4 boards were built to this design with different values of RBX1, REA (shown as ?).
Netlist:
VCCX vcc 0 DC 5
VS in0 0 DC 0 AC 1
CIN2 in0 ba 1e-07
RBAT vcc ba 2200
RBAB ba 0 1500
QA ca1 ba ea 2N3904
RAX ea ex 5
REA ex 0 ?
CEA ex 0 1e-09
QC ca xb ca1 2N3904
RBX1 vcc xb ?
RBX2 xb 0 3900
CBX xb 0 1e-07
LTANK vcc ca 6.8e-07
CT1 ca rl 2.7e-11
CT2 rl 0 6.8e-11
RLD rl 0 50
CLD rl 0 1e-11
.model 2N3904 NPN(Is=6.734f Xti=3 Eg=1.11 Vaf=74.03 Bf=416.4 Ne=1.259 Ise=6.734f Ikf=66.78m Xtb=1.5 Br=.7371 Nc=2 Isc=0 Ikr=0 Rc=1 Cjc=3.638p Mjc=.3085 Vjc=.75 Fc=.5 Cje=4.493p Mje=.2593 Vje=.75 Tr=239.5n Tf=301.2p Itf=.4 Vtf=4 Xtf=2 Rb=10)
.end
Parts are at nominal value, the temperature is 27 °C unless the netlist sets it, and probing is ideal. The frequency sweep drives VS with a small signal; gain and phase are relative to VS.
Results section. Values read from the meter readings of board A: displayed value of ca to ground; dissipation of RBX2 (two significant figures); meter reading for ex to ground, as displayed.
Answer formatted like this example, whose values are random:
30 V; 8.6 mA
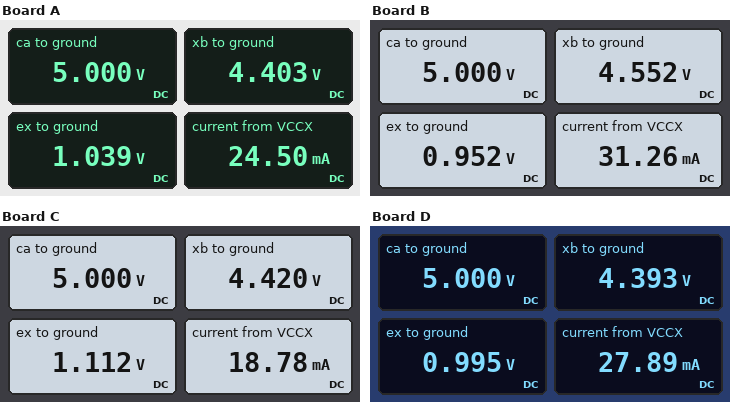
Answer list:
5.000 V; 5.0 mW; 1.039 V
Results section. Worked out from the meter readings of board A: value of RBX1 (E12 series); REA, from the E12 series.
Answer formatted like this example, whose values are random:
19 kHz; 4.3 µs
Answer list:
470 Ω; 47 Ω
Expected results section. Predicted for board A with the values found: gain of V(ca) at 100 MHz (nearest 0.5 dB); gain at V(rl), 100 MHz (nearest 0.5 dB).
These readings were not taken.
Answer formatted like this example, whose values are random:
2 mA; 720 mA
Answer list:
20.5 dB; 8.5 dB
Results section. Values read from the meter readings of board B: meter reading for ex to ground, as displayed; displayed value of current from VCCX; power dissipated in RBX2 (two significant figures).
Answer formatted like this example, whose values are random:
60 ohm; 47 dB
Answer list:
0.952 V; 31.26 mA; 5.3 mW
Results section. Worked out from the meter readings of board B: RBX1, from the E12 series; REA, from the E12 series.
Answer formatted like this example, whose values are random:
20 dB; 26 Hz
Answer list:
330 Ω; 33 Ω
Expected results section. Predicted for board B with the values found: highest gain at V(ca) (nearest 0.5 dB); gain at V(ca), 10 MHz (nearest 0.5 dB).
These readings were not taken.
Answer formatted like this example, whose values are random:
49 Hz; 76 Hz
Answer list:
44.0 dB; 8.0 dB
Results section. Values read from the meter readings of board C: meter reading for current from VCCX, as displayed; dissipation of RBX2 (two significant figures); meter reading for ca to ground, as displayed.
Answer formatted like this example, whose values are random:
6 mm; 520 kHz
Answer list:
18.78 mA; 5.0 mW; 5.000 V
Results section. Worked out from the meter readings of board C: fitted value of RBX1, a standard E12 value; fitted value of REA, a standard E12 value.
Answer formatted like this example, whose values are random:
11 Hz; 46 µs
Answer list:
470 Ω; 68 Ω
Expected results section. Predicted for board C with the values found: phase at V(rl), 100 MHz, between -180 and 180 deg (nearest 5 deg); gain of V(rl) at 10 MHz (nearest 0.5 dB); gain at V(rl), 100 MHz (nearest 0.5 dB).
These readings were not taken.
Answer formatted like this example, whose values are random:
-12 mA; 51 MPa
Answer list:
90 deg; -14.0 dB; 8.0 dB
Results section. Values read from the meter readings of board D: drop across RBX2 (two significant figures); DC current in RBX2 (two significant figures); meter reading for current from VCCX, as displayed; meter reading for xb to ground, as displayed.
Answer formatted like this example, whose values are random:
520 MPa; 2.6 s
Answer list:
4.4 V; 1.1 mA; 27.89 mA; 4.393 V
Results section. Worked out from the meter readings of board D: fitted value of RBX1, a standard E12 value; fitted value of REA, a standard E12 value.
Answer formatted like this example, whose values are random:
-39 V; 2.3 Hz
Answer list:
470 Ω; 39 Ω
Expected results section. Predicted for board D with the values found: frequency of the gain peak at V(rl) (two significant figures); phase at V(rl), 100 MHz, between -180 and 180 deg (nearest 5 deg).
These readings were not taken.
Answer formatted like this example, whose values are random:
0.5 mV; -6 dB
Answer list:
38 MHz; 85 deg
